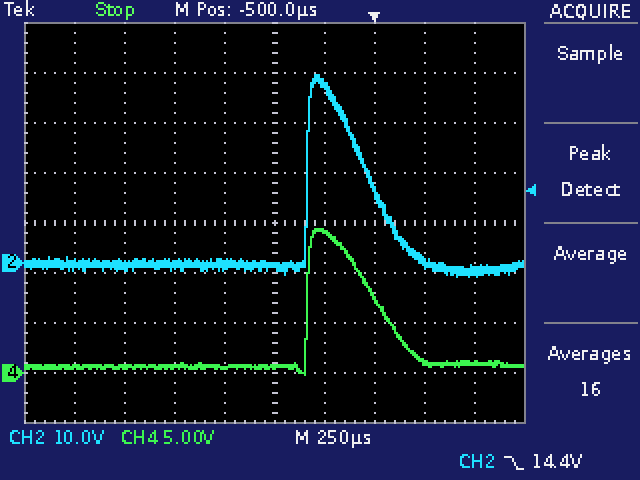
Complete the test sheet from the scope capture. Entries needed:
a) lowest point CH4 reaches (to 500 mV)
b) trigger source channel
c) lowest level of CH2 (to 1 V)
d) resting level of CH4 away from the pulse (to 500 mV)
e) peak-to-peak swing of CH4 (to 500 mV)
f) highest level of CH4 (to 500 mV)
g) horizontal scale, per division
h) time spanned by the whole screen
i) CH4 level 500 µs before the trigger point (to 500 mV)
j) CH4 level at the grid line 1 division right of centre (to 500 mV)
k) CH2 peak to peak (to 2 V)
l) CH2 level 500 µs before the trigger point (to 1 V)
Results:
0.0 V
CH2
-3 V
500 mV
14.5 V
14.5 V
250 µs
2.5 ms
500 mV
14.0 V
40 V
-1 V
